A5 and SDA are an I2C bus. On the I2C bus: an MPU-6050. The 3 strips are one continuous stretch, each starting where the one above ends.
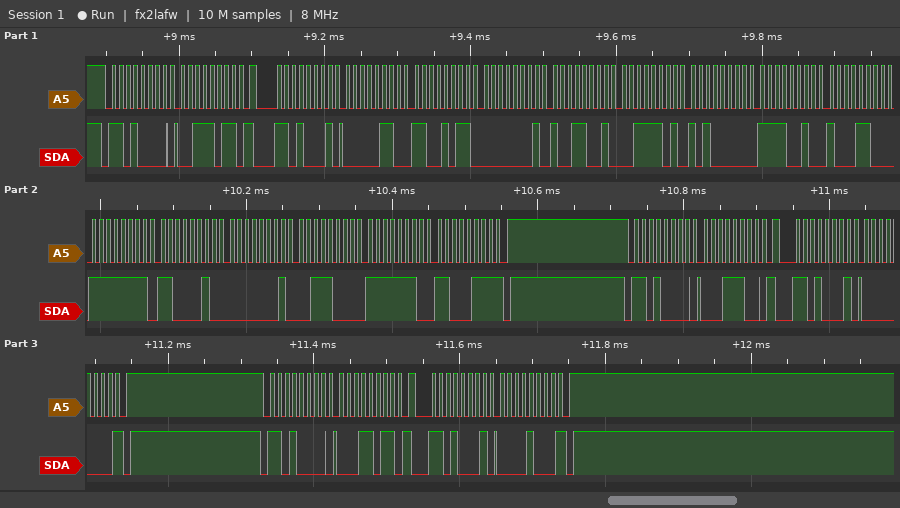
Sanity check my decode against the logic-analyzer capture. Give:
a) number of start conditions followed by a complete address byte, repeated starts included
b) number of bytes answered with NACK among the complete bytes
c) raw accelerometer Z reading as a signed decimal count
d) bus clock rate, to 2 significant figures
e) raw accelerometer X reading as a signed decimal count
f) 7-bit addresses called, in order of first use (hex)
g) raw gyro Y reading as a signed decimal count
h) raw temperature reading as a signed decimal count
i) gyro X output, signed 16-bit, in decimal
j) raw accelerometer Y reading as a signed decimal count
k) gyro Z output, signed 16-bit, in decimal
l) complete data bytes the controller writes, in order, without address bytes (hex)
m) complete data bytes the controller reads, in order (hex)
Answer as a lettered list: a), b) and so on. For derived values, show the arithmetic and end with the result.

a) 6
b) 3
c) 0x3DA0 = 15776
d) 100 kHz
e) 0x06CB = 1739
f) 0x68
g) 0x0138 = 312
h) 0xF28C = -3444
i) 0xFFC2 = -62
j) 0x0199 = 409
k) 0xFEC7 = -313
l) 3B 1C 1B
m) 06 CB 01 99 3D A0 F2 8C FF C2 01 38 FE C7 00 08
